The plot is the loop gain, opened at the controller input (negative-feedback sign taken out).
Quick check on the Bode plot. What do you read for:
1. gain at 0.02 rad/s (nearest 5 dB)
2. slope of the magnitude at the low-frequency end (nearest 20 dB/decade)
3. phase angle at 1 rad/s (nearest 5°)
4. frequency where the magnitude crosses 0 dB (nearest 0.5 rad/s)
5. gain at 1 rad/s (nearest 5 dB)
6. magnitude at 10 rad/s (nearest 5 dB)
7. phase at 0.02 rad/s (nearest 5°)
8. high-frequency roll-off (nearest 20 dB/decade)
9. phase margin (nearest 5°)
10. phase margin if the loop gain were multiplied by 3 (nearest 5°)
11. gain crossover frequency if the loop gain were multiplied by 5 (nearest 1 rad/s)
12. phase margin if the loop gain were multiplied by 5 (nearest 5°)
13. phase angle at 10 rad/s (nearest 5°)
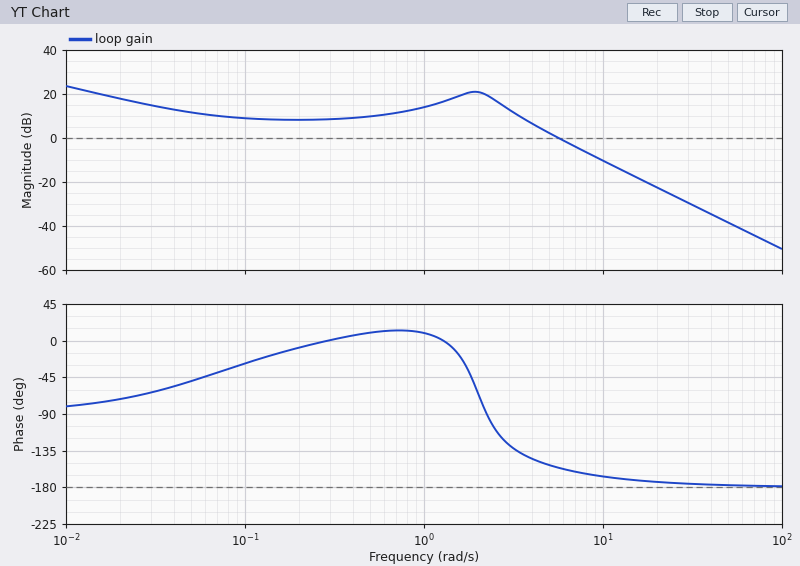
20 dB
-20 dB/decade
10°
5.5 rad/s
15 dB
-10 dB
-70°
-40 dB/decade
25°
15°
12 rad/s
10°
-165°
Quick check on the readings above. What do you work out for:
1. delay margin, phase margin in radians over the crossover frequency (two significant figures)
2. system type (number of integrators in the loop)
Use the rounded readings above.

0.079 s
1
